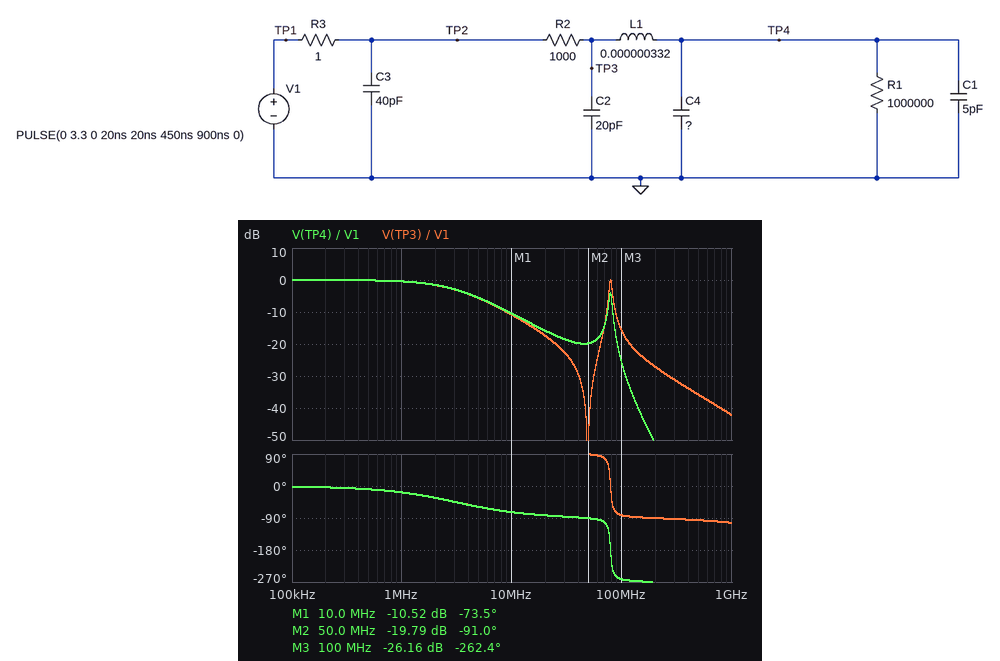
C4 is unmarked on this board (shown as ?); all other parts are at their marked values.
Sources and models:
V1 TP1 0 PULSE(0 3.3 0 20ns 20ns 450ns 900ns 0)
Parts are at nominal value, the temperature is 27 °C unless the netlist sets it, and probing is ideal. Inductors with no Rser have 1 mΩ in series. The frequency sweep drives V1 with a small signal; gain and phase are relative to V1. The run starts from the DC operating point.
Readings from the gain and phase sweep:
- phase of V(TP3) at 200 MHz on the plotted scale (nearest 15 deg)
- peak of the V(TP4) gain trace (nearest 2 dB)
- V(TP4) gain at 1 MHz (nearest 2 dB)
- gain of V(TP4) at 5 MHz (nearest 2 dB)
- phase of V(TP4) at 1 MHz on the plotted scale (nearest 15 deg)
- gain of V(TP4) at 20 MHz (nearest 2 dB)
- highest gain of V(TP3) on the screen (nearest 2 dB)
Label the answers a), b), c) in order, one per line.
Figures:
a) -90 deg
b) 0 dB
c) 0 dB
d) -6 dB
e) -15 deg
f) -16 dB
g) 0 dB
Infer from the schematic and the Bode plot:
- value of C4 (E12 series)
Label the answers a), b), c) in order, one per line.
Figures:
a) 27 pF
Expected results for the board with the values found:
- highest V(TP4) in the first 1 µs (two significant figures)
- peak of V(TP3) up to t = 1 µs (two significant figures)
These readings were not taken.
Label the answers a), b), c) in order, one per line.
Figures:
a) 3.3 V
b) 3.3 V
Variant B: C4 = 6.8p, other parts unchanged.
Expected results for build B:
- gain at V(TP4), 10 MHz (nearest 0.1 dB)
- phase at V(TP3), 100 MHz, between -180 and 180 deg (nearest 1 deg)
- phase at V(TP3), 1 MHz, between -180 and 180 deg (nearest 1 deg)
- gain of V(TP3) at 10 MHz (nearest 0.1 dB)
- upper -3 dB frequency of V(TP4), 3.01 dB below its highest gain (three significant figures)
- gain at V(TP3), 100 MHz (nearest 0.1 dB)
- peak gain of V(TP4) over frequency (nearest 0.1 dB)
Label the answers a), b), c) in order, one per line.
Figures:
a) -6.9 dB
b) 43 deg
c) -11 deg
d) -7.0 dB
e) 103 MHz
f) -3.0 dB
g) 4.6 dB
